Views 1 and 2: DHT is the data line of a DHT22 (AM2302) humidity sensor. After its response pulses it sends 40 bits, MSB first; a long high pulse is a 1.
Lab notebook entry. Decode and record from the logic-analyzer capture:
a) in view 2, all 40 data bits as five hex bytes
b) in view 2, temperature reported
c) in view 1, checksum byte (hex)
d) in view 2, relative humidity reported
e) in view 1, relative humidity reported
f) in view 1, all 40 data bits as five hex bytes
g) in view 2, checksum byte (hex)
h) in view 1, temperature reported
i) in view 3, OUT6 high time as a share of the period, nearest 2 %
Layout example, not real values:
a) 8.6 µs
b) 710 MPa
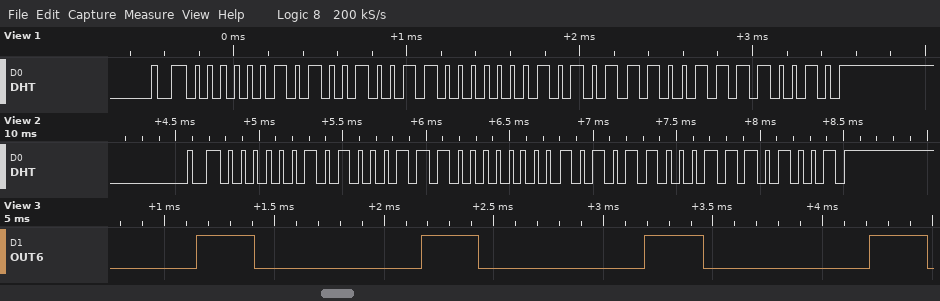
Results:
a) 02 8E 01 58 E9
b) 34.4 °C
c) 0xF2
d) 65.4 %
e) 65.9 %
f) 02 93 01 5C F2
g) 0xE9
h) 34.8 °C
i) 26 %
